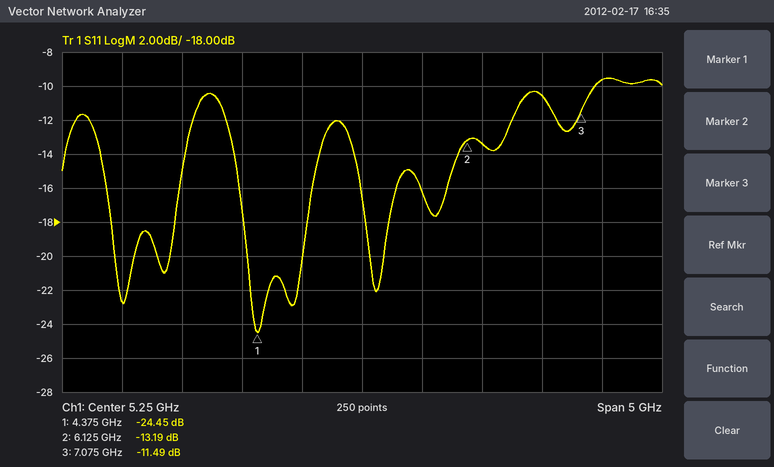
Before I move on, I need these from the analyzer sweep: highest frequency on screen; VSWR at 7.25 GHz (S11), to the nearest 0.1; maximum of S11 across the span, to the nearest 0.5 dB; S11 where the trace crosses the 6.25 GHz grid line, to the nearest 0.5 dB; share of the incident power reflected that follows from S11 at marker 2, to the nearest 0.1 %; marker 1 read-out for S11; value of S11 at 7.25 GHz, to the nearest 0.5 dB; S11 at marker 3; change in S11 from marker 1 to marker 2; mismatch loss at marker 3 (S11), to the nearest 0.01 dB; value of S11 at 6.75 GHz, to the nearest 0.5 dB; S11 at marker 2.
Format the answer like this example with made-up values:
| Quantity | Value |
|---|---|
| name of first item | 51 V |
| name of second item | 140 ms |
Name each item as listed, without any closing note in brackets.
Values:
| Quantity | Value |
|---|---|
| highest frequency on screen | 7.75 GHz |
| VSWR at 7.25 GHz (S11), to the nearest 0.1 | 2.0 |
| maximum of S11 across the span, to the nearest 0.5 dB | -9.5 dB |
| S11 where the trace crosses the 6.25 GHz grid line, to the nearest 0.5 dB | -13.5 dB |
| share of the incident power reflected that follows from S11 at marker 2, to the nearest 0.1 % | 4.8 % |
| marker 1 read-out for S11 | -24.45 dB |
| value of S11 at 7.25 GHz, to the nearest 0.5 dB | -9.5 dB |
| S11 at marker 3 | -11.49 dB |
| change in S11 from marker 1 to marker 2 | 11.26 dB |
| mismatch loss at marker 3 (S11), to the nearest 0.01 dB | 0.32 dB |
| value of S11 at 6.75 GHz, to the nearest 0.5 dB | -10.5 dB |
| S11 at marker 2 | -13.19 dB |
